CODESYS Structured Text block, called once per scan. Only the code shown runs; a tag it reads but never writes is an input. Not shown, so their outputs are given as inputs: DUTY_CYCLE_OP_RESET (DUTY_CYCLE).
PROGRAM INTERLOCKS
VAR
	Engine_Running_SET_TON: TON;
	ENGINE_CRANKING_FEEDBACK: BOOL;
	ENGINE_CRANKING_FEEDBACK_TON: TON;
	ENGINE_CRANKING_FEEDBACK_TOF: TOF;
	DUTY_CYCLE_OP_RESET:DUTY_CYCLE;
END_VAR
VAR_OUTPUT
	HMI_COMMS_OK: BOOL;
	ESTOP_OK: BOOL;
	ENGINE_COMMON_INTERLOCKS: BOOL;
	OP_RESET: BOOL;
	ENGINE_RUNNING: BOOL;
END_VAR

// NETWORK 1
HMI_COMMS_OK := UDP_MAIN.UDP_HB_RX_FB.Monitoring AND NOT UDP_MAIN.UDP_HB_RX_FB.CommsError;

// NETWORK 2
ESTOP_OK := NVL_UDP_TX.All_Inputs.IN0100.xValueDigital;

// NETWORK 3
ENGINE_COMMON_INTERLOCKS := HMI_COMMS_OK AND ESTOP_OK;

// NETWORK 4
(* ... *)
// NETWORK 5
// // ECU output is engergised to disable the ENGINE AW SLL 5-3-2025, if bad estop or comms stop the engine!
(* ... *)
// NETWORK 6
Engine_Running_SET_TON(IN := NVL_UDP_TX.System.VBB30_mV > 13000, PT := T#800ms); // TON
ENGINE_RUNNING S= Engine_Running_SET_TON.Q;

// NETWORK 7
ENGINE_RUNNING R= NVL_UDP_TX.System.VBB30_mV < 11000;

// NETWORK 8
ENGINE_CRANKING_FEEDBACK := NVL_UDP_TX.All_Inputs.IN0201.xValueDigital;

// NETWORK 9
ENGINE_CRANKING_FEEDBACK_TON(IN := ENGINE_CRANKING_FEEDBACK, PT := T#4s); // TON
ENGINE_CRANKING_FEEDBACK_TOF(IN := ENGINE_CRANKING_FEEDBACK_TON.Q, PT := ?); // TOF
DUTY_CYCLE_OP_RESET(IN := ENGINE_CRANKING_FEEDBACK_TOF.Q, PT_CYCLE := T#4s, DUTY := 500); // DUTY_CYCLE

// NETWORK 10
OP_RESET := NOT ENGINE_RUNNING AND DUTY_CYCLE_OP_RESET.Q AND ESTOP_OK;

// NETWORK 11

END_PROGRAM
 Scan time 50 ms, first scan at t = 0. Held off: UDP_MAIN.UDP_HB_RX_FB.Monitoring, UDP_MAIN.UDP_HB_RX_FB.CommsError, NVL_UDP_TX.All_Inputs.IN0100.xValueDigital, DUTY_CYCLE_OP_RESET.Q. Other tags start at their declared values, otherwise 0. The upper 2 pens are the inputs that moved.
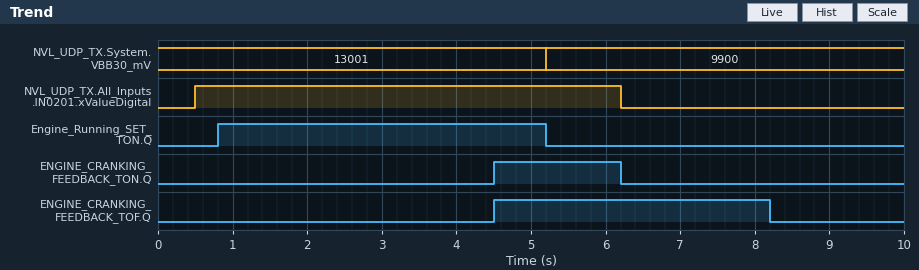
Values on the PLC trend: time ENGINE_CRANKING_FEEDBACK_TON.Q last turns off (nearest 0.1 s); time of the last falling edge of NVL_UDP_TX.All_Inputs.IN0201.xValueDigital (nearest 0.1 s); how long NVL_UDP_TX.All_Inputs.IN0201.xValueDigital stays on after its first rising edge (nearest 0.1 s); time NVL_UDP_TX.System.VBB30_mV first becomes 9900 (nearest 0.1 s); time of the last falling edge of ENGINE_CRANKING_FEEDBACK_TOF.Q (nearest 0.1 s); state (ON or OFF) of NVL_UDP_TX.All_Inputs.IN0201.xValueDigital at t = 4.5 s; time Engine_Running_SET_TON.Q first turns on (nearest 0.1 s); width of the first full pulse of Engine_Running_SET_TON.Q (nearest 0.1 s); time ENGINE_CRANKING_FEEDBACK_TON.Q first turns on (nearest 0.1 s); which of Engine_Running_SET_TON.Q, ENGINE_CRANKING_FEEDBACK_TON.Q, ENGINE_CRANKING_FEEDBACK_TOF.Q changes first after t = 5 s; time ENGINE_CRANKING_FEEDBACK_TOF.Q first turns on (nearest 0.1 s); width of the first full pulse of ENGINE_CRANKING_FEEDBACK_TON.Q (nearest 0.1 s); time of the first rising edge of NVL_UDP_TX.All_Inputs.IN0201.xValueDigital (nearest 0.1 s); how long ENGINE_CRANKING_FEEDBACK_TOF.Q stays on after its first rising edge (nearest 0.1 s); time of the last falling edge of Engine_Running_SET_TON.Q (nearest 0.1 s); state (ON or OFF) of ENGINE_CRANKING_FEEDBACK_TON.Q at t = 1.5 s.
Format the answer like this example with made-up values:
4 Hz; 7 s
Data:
6.2 s; 6.2 s; 5.7 s; 5.2 s; 8.2 s; ON; 0.8 s; 4.4 s; 4.5 s; Engine_Running_SET_TON.Q; 4.5 s; 1.7 s; 0.5 s; 3.7 s; 5.2 s; OFF
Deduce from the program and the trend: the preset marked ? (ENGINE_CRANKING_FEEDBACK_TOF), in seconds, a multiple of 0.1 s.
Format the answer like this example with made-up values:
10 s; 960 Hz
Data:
2.0 s
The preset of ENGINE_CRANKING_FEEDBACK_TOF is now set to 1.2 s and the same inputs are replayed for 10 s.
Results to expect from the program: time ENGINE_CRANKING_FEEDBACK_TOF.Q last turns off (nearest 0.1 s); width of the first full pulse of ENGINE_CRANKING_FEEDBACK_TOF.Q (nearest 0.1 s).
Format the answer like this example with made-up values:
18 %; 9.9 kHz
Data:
7.4 s; 2.9 s
